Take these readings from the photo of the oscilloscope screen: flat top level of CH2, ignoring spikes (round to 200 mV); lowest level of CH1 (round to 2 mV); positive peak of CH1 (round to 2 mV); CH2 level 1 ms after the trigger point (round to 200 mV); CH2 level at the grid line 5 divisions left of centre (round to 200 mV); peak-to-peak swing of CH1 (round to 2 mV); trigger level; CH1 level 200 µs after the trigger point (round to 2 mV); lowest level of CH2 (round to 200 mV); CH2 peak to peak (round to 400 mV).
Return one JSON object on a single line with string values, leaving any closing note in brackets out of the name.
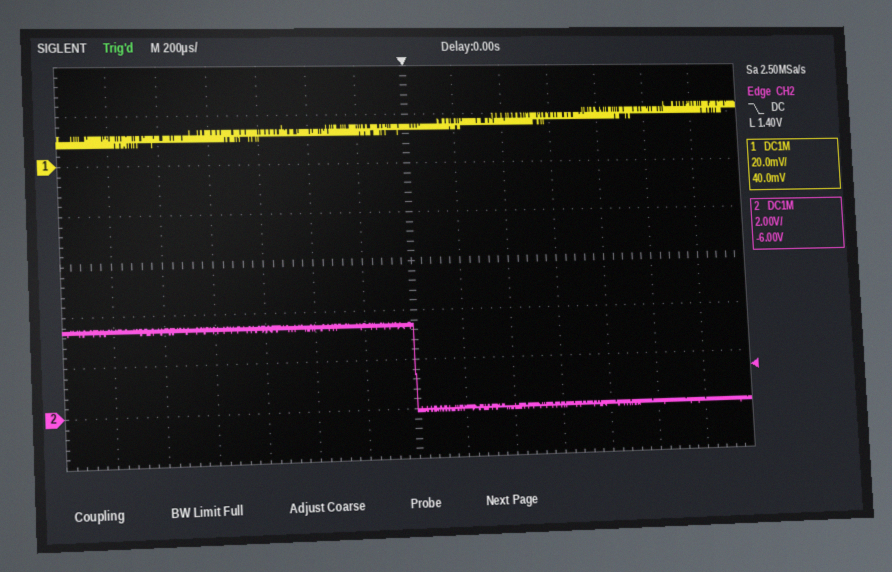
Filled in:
{"flat top level of CH2, ignoring spikes": "3.4 V", "lowest level of CH1": "8 mV", "positive peak of CH1": "24 mV", "CH2 level 1 ms after the trigger point": "0.0 V", "CH2 level at the grid line 5 divisions left of centre": "3.4 V", "peak-to-peak swing of CH1": "16 mV", "trigger level": "1.40 V", "CH1 level 200 µs after the trigger point": "16 mV", "lowest level of CH2": "0.0 V", "CH2 peak to peak": "3.6 V"}
